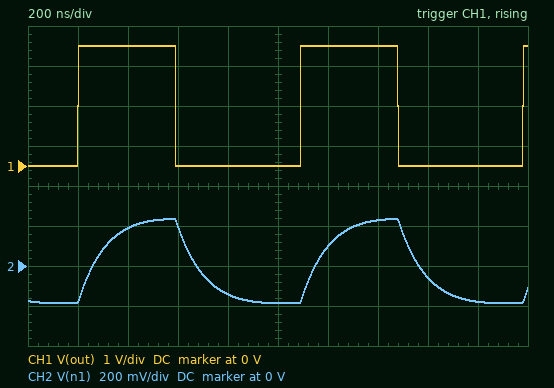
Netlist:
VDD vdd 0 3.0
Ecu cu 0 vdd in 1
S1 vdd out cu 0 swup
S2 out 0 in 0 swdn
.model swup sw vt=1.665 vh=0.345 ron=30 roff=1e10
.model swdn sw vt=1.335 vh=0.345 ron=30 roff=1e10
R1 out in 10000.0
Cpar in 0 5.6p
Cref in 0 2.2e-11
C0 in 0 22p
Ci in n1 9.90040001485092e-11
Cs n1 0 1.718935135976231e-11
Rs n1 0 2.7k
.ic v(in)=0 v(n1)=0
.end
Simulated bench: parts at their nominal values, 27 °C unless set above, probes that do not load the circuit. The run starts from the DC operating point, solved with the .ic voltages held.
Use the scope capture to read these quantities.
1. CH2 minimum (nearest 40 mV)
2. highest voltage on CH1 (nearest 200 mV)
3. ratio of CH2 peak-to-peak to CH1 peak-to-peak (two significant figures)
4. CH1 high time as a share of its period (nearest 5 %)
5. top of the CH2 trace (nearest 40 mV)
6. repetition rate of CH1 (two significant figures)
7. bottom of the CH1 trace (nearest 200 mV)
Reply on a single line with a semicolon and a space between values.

-200 mV; 3.0 V; 0.14; 45 %; 240 mV; 1.1 MHz; 0 V
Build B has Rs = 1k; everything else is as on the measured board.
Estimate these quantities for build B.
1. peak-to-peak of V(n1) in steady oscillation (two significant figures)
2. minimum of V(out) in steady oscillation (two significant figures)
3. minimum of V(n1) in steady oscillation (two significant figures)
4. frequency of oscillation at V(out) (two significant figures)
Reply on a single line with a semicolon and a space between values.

200 mV; 3.0 mV; -90 mV; 810 kHz
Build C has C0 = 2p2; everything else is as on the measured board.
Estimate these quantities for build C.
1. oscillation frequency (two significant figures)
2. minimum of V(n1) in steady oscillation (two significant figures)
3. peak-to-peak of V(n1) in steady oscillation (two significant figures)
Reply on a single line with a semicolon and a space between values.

1.6 MHz; -210 mV; 470 mV
